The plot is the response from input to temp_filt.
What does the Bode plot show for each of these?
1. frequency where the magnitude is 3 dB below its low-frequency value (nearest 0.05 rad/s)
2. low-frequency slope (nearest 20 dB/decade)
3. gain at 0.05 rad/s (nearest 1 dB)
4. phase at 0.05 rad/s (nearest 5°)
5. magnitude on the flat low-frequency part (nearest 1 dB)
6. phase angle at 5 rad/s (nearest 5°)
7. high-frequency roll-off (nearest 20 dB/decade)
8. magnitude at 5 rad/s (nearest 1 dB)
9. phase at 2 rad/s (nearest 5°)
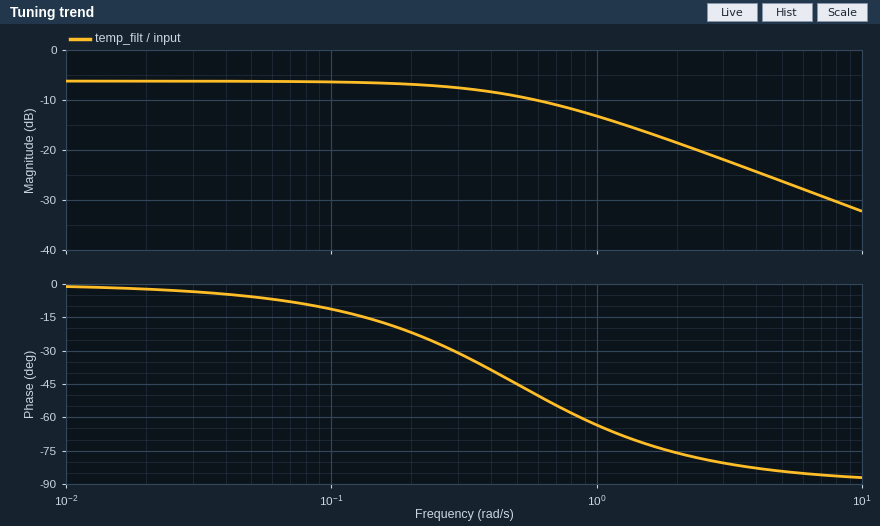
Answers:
0.50 rad/s
0 dB/decade
-6 dB
-5°
-6 dB
-85°
-20 dB/decade
-26 dB
-75°
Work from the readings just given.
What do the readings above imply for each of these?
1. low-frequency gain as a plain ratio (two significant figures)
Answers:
0.50
